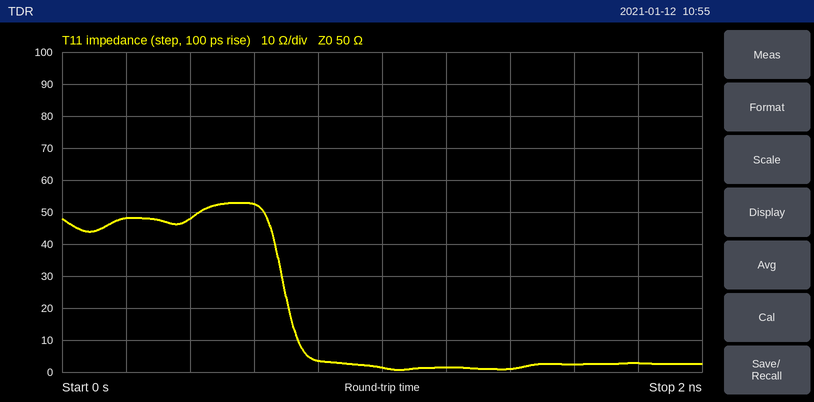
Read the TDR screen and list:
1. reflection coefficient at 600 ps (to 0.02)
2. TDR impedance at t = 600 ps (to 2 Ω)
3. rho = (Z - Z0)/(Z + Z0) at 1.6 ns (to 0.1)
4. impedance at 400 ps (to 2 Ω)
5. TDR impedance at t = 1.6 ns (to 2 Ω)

+0.02
52 Ω
-0.9
48 Ω
2 Ω
